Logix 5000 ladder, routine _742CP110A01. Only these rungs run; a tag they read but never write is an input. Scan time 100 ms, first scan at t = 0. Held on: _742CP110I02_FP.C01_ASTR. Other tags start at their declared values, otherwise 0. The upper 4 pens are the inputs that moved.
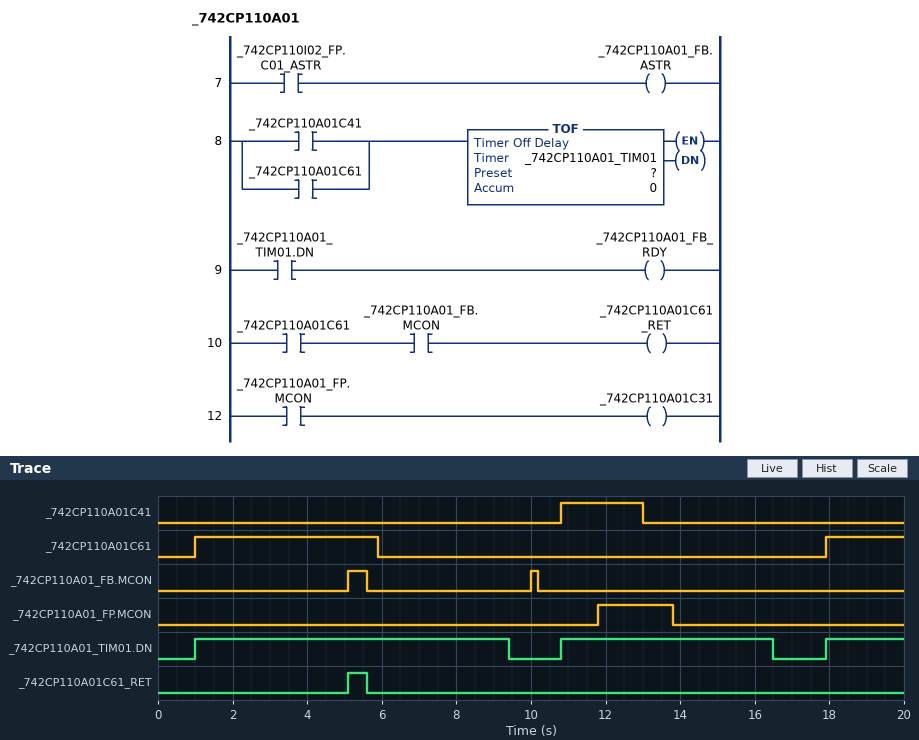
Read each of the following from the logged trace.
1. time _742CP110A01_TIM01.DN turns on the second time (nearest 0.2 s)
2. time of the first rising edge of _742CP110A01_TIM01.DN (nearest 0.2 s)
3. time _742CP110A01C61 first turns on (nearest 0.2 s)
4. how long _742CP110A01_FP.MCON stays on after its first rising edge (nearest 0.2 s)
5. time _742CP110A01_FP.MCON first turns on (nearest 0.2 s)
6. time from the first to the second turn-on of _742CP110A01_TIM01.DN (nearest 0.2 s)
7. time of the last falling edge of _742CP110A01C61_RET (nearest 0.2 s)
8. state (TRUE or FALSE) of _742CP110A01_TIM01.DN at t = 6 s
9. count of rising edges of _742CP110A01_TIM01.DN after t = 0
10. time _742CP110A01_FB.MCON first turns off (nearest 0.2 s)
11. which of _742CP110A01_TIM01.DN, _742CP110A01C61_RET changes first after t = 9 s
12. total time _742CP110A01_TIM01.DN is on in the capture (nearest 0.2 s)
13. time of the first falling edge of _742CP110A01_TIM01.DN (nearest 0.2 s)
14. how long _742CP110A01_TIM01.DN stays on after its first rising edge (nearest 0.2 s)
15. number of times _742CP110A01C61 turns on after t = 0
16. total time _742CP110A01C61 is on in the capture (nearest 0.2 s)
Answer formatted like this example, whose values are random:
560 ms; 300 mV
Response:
10.8 s; 1.0 s; 1.0 s; 2.0 s; 11.8 s; 9.8 s; 5.6 s; TRUE; 3; 5.6 s; _742CP110A01_TIM01.DN; 16.2 s; 9.4 s; 8.4 s; 2; 7.0 s
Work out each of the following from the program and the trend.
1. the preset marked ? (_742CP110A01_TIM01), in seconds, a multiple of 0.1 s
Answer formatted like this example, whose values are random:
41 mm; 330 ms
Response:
3.5 s
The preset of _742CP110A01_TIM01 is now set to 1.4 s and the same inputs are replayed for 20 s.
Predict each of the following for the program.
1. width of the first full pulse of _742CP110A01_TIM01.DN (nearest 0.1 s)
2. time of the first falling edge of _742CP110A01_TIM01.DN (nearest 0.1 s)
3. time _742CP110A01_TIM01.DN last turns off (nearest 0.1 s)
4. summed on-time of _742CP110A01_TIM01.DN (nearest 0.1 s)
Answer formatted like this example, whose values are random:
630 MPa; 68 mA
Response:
6.3 s; 7.3 s; 14.4 s; 12.0 s
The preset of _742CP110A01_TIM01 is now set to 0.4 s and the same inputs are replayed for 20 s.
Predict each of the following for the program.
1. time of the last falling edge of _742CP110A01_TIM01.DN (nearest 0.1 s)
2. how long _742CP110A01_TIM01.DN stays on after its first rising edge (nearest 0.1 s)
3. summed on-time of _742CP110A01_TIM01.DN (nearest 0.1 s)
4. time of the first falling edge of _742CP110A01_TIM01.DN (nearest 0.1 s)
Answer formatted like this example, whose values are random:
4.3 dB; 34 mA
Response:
13.4 s; 5.3 s; 10.0 s; 6.3 s
